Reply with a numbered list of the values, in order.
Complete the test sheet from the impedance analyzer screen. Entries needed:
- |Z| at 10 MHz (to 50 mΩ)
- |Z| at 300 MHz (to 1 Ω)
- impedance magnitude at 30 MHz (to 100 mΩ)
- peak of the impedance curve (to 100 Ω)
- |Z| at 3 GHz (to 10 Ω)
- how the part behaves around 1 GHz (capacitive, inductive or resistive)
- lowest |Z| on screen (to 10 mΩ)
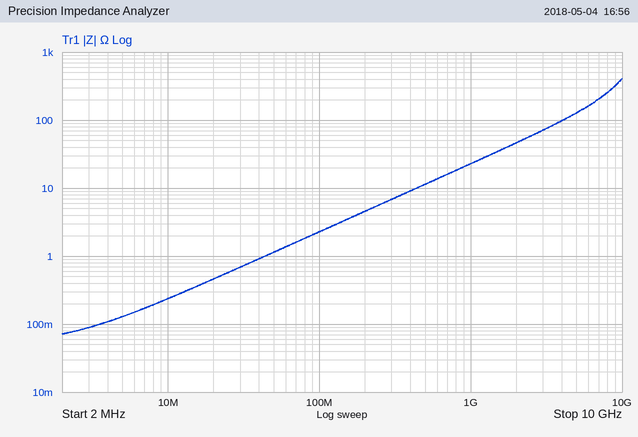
1. 250 mΩ
2. 7 Ω
3. 700 mΩ
4. 400 Ω
5. 70 Ω
6. inductive
7. 70 mΩ
